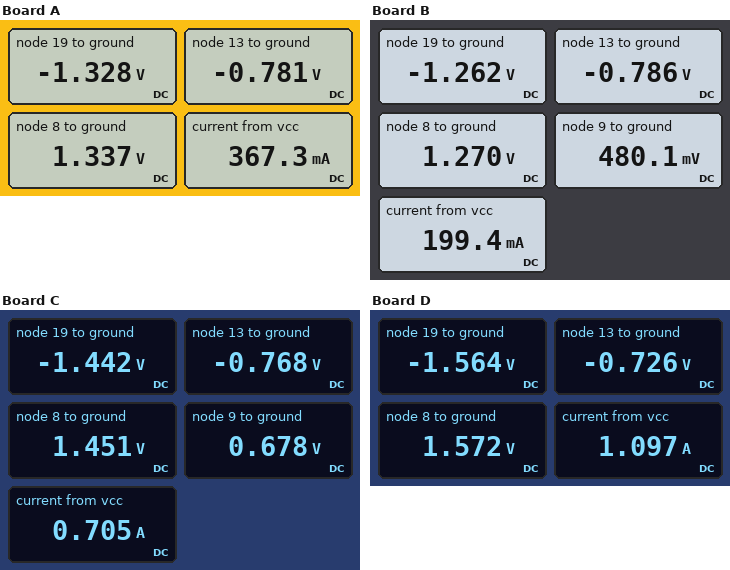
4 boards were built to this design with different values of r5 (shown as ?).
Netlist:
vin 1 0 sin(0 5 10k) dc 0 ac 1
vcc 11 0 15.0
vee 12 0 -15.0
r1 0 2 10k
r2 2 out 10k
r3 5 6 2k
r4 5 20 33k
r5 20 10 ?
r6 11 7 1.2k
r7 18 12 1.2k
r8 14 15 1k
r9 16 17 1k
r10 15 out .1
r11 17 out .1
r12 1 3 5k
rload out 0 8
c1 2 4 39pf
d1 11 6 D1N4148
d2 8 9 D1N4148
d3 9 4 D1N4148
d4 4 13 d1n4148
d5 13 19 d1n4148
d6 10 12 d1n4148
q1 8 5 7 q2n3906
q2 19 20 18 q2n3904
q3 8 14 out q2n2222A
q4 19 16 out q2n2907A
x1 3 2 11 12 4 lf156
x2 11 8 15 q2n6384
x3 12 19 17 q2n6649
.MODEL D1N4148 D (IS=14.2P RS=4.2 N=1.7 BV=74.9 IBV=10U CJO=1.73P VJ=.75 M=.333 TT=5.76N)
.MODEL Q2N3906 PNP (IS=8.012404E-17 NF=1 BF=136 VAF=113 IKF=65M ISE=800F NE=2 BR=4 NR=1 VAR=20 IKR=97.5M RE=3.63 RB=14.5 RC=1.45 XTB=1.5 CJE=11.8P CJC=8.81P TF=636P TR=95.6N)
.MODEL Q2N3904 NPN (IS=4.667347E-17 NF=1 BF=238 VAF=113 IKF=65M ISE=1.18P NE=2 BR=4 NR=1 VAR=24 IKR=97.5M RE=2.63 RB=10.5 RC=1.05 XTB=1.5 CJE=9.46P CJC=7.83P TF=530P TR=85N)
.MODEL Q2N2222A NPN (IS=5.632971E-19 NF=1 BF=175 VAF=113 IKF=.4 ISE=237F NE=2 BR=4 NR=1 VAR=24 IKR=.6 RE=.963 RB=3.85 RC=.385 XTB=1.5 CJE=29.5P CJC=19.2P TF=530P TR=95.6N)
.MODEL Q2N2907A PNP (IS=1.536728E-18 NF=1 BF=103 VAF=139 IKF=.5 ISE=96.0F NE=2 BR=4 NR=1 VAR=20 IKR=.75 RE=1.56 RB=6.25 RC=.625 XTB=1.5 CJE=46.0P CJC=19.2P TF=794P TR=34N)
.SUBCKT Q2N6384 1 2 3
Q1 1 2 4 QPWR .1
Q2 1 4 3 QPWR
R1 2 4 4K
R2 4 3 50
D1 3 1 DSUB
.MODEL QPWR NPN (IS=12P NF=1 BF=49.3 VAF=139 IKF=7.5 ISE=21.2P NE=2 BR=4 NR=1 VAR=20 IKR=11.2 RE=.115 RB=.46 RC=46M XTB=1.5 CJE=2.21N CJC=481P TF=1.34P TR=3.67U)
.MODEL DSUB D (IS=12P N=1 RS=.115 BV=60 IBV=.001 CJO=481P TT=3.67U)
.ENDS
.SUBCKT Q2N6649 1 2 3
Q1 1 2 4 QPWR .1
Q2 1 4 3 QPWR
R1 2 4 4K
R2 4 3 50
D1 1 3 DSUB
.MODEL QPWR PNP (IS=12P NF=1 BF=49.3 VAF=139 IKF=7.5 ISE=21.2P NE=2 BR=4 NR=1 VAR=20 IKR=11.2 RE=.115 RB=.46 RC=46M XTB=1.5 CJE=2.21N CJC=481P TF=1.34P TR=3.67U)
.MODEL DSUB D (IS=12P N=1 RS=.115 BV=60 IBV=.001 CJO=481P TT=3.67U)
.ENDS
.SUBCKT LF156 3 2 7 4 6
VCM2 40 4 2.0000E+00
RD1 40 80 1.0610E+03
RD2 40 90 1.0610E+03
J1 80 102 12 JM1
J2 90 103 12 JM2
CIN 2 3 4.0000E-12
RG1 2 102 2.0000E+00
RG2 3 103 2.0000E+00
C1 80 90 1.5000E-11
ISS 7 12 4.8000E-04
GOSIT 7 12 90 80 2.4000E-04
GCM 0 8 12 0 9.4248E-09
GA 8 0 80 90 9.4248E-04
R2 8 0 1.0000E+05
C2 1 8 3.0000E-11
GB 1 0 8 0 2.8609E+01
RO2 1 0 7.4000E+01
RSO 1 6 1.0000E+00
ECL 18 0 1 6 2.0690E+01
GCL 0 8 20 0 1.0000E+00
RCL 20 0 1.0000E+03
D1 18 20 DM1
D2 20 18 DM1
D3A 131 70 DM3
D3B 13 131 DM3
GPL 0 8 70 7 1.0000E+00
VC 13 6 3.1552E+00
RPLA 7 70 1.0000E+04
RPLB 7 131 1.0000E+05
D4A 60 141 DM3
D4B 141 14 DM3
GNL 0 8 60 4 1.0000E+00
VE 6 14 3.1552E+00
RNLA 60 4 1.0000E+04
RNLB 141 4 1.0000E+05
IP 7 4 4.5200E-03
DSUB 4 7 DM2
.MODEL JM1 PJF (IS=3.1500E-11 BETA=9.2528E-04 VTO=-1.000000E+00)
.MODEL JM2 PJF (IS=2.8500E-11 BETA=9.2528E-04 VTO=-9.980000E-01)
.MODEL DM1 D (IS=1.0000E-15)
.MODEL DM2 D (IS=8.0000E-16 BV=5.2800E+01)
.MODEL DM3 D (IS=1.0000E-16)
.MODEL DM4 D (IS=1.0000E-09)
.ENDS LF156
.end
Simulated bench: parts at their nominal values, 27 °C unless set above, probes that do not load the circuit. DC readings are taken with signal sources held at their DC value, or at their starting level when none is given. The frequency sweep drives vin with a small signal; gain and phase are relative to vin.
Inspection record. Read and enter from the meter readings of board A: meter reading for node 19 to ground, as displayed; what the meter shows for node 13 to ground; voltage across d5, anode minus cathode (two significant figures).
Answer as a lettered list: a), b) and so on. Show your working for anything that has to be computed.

a) -1.328 V
b) -0.781 V
c) -781 mV - (-1.328 V) = 550 mV
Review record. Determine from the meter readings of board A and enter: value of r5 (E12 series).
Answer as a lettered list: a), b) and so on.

a) 820 Ω
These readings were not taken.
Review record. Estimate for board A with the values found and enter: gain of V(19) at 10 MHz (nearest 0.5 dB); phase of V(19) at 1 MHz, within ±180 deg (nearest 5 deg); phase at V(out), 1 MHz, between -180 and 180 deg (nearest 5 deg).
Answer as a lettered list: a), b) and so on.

a) -23.5 dB
b) -50 deg
c) -40 deg
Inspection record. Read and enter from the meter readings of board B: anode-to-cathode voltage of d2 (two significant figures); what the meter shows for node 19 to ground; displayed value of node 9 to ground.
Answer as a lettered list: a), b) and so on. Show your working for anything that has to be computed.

a) 1.27 V - 480.1 mV = 790 mV
b) -1.262 V
c) 480.1 mV
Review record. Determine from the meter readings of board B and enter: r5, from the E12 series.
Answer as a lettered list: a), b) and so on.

a) 680 Ω
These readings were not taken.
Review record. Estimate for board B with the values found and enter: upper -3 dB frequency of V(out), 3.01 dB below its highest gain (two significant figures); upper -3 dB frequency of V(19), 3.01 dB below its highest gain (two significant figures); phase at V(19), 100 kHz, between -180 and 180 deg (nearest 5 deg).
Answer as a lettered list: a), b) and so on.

a) 510 kHz
b) 490 kHz
c) -10 deg
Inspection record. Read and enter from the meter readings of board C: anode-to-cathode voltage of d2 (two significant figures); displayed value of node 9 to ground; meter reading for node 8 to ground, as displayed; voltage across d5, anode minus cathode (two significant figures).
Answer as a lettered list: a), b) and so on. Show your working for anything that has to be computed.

a) 1.451 V - 678 mV = 770 mV
b) 0.678 V
c) 1.451 V
d) -768 mV - (-1.442 V) = 670 mV
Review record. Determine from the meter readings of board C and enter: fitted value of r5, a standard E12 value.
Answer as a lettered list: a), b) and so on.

a) 1.2 kΩ
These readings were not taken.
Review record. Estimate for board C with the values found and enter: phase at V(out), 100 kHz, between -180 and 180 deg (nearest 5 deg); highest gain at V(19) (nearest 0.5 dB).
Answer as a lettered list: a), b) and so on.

a) -10 deg
b) 6.0 dB
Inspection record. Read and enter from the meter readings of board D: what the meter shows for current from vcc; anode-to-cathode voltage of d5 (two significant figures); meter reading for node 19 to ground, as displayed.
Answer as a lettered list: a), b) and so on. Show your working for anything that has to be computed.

a) 1.097 A
b) -726 mV - (-1.564 V) = 840 mV
c) -1.564 V
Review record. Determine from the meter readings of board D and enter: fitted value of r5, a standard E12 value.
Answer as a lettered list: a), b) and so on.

a) 5.6 kΩ
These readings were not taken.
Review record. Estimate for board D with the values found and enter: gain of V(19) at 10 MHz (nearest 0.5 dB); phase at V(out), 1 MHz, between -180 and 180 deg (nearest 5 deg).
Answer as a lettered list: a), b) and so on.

a) -17.0 dB
b) -35 deg
